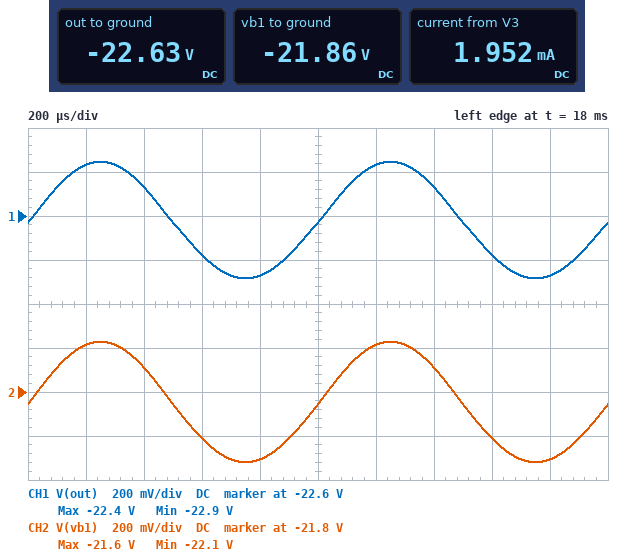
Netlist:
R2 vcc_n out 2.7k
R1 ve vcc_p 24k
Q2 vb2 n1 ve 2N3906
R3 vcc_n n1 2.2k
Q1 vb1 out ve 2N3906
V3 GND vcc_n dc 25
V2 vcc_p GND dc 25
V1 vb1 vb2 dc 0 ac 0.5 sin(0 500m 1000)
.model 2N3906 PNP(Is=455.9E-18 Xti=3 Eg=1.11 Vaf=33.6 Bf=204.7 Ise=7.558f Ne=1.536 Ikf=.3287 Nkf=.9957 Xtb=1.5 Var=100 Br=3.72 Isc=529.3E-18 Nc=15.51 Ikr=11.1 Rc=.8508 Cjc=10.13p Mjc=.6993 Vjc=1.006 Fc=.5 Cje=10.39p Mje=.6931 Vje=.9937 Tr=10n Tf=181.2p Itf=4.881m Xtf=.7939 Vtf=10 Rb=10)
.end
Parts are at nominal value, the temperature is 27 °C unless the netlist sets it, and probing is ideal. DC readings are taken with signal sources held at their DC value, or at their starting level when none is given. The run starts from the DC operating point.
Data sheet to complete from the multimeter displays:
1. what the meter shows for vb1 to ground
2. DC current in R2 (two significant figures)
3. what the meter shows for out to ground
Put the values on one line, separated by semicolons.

-21.86 V; 880 µA; -22.63 V
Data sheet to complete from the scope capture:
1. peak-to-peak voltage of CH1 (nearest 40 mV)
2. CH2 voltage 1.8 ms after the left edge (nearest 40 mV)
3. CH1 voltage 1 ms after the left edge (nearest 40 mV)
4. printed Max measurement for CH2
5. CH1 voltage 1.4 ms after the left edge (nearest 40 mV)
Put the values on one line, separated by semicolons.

520 mV; -22.12 V; -22.64 V; -21.6 V; -22.48 V
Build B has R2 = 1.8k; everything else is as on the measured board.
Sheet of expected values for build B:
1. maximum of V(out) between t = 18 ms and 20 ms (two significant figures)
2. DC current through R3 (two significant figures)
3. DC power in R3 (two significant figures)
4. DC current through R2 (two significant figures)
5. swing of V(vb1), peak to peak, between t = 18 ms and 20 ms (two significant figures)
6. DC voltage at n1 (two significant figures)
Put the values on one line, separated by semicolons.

-23 V; 890 µA; 1.7 mW; 1.1 mA; 450 mV; -23 V
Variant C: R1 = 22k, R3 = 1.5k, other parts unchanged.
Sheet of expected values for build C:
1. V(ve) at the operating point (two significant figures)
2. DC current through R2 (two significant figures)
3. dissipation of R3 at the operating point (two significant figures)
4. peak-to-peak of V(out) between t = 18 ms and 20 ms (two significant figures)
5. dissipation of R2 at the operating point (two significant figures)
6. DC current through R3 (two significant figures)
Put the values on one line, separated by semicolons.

-22 V; 770 µA; 2.8 mW; 610 mV; 1.6 mW; 1.4 mA
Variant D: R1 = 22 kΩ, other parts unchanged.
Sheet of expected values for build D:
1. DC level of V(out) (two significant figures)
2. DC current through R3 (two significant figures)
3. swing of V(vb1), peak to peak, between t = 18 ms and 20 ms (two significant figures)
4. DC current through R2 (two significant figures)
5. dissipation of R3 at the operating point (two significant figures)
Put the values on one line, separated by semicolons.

-22 V; 1.2 mA; 550 mV; 950 µA; 3.0 mW
